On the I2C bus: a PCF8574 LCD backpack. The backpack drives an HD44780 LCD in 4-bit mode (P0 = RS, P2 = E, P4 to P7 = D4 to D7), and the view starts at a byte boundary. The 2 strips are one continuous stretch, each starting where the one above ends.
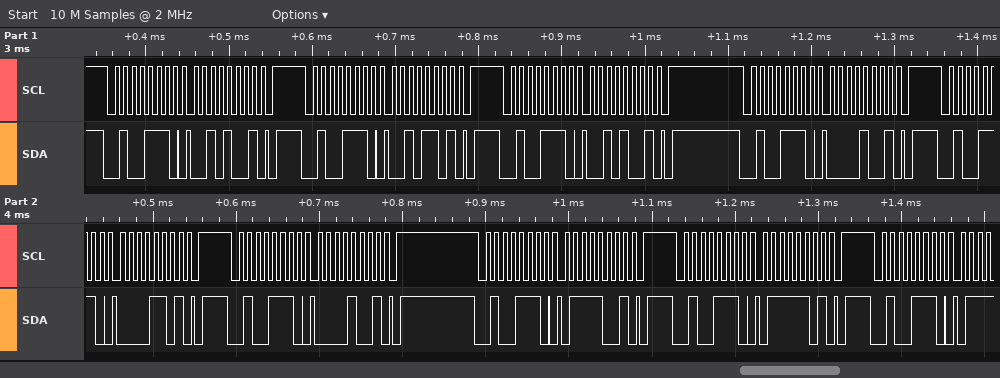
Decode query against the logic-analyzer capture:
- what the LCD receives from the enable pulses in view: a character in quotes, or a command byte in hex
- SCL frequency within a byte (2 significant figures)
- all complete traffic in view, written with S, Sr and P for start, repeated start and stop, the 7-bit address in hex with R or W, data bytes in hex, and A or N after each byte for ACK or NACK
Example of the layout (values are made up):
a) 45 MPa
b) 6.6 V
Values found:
a) ' '
b) 100 kHz
c) S 27W A 29 A P S 27W A 2D A P S 27W A 29 A P S 27W A 09 A P S 27W A 0D A P S 27W A 09 A P S 27W A 79 A P S 27W A 7D A P S 27W A
